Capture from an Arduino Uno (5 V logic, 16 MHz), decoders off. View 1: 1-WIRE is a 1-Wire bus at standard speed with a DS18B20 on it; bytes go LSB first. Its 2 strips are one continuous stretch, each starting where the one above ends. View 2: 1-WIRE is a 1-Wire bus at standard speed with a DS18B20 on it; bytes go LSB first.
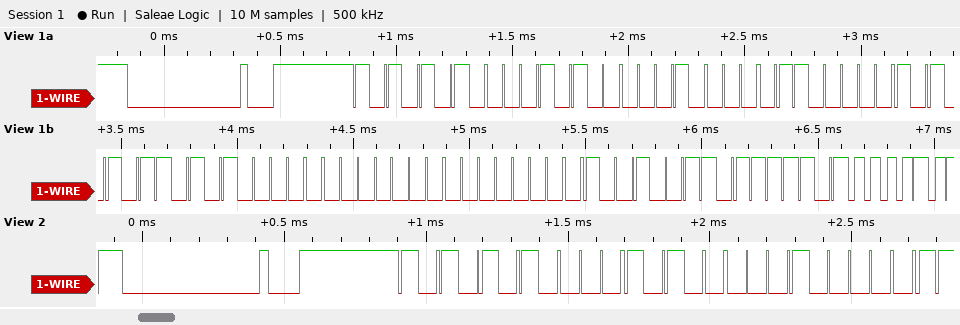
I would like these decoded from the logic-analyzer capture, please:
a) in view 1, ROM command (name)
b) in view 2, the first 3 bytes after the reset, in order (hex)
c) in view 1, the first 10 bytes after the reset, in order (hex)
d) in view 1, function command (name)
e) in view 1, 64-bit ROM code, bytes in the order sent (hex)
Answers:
Match ROM
55 28 08
55 28 08 06 D5 0A 00 00 C9 BE
Read Scratchpad
28 08 06 D5 0A 00 00 C9
